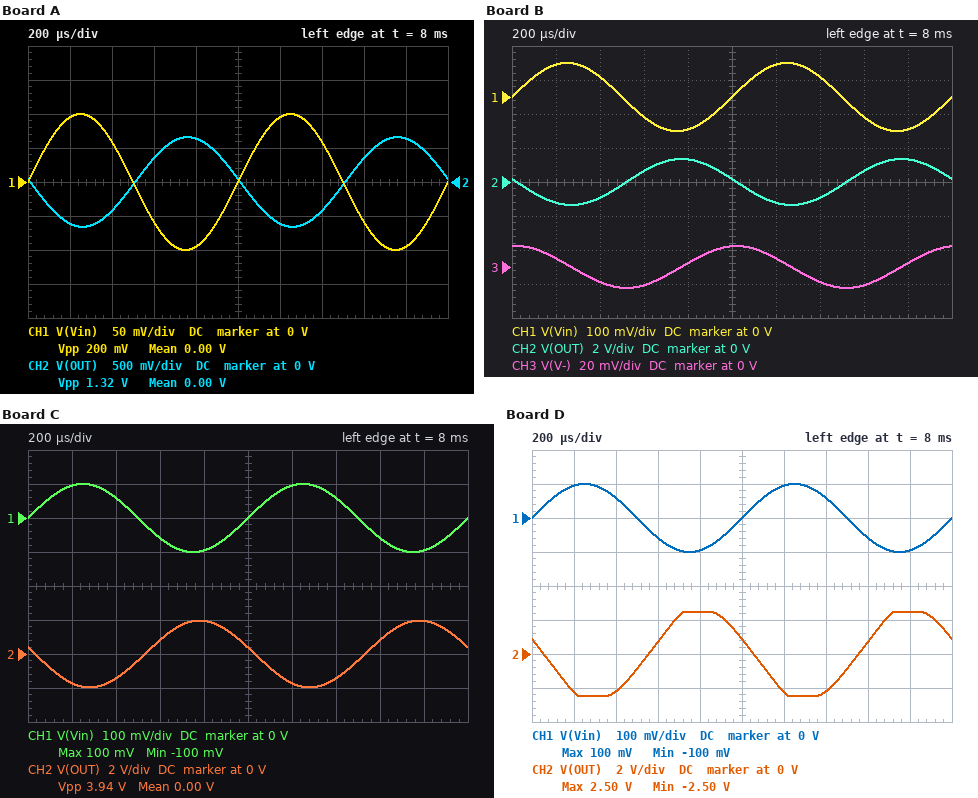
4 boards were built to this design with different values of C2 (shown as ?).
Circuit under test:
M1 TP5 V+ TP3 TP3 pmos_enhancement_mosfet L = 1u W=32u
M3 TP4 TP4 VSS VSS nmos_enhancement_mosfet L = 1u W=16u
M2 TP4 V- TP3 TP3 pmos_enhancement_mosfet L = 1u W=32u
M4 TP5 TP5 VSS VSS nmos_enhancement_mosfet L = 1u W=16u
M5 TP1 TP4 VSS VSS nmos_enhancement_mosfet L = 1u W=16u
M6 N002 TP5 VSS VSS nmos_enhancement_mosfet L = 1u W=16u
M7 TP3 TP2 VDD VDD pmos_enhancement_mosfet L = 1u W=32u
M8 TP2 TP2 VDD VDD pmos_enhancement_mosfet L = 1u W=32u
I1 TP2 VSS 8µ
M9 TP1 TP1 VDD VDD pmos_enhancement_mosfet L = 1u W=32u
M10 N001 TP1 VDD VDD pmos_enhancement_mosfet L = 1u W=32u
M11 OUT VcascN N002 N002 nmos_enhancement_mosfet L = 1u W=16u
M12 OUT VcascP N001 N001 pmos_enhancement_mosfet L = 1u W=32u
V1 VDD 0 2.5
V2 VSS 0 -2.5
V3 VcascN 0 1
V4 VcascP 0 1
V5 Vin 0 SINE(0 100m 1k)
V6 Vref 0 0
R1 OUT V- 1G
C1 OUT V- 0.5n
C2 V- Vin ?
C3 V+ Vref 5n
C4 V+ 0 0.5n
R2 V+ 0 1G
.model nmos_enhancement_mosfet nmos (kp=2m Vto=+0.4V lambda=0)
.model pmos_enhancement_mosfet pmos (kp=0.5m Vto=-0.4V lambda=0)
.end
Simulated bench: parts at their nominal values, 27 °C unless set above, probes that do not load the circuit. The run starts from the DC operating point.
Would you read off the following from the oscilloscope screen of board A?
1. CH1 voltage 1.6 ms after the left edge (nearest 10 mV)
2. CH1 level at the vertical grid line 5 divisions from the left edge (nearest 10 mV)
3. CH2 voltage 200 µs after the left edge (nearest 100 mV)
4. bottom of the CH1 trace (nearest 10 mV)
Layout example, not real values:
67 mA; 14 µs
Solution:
-60 mV; 0 V; -600 mV; -100 mV
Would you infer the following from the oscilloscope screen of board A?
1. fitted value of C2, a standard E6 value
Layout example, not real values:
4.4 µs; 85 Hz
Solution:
3.3 nF
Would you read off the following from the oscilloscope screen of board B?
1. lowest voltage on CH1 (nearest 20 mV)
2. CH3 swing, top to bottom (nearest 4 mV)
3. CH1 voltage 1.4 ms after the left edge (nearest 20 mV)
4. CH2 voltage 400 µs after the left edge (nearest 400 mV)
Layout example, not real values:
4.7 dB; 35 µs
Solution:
-100 mV; 24 mV; 60 mV; -800 mV
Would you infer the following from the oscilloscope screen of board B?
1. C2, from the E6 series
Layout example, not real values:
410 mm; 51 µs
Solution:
6.8 nF
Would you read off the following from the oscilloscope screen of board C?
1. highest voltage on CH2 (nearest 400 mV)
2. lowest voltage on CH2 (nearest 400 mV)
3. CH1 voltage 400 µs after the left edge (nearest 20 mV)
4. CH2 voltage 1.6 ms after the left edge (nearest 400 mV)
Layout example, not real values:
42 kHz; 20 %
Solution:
2.0 V; -2.0 V; 60 mV; 800 mV
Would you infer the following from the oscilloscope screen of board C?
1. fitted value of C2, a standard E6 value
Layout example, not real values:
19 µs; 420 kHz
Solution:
10 nF
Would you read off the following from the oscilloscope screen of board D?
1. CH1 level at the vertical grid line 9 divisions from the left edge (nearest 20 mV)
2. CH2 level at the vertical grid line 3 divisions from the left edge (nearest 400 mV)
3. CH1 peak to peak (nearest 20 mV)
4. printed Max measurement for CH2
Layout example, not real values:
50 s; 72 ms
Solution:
-100 mV; 800 mV; 200 mV; 2.50 V
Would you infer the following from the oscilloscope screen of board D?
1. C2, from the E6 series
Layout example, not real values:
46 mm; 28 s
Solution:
15 nF
